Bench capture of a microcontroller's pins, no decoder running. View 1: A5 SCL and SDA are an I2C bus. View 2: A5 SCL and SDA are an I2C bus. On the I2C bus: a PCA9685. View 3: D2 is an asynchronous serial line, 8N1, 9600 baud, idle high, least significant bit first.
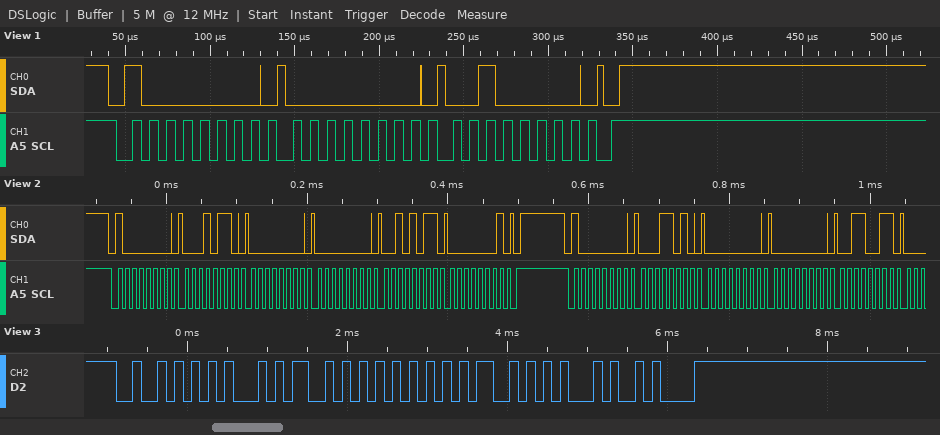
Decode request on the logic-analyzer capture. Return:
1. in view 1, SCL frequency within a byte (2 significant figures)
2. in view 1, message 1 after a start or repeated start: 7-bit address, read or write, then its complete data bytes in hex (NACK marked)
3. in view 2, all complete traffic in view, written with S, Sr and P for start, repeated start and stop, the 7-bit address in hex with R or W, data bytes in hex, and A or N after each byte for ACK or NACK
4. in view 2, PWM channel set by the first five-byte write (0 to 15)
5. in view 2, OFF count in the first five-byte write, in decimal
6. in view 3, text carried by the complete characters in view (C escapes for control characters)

100 kHz
0x40 write: 00 20
S 40W A 16 A 00 A 00 A 2B A 01 A P S 40W A 1A A 00 A 00 A 33 A
4
299
"RESUME\n"
